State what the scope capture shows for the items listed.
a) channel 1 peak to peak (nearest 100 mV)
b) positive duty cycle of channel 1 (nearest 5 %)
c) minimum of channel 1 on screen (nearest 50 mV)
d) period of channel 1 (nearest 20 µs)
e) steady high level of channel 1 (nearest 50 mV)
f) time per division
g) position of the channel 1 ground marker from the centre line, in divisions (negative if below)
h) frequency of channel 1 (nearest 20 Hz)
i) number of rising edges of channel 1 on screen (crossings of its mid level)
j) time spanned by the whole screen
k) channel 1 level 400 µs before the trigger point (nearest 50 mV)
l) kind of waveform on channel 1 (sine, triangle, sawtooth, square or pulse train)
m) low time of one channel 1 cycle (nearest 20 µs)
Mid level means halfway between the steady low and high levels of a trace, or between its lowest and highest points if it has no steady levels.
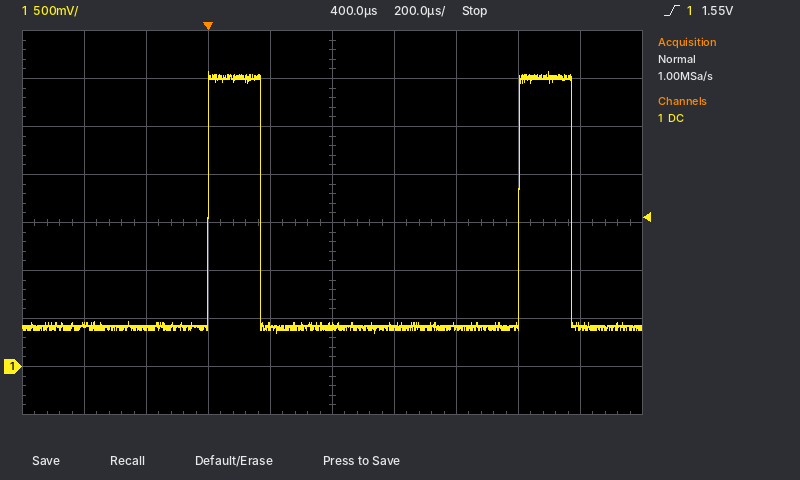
2.70 V
15 %
350 mV
1.00 ms
3.00 V
200 µs
-3.0 div
1.00 kHz
2
2 ms
450 mV
pulse train
840 µs
